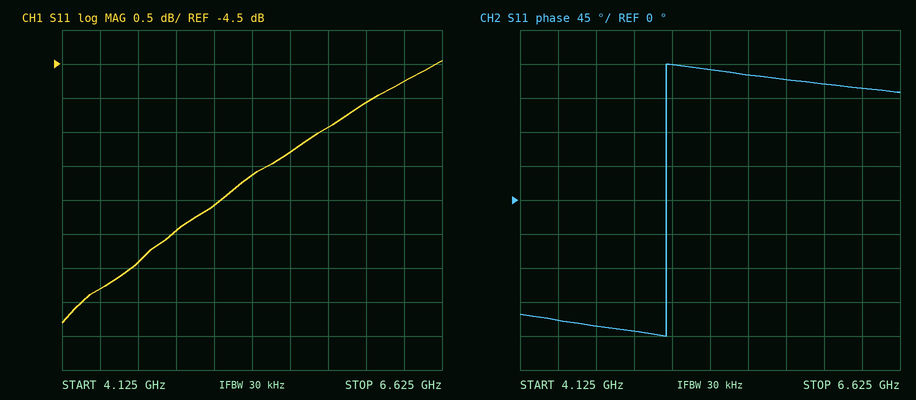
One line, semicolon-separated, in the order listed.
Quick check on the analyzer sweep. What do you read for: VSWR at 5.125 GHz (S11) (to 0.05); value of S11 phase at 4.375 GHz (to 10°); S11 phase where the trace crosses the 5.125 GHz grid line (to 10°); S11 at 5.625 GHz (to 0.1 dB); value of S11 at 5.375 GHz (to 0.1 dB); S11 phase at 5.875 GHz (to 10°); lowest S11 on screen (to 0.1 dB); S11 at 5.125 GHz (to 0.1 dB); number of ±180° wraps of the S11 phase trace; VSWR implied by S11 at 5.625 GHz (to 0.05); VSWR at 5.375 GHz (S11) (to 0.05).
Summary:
2.75; -160°; 180°; -5.8 dB; -6.1 dB; 160°; -8.3 dB; -6.6 dB; 1; 3.10; 2.95
